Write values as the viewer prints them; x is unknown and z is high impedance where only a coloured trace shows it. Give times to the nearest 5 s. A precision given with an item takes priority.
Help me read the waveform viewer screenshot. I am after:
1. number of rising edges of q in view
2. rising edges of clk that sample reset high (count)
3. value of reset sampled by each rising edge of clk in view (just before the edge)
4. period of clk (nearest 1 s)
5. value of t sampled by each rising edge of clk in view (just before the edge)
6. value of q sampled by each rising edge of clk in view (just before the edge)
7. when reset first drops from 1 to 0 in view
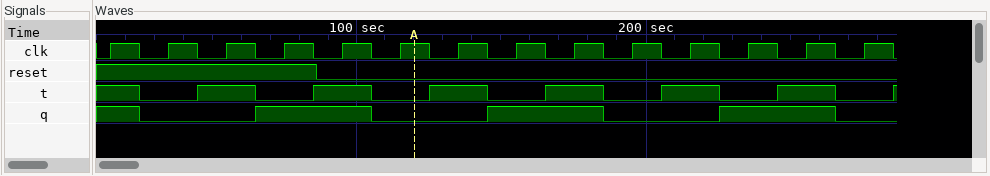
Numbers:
3
4
1 1 1 1 0 0 0 0 0 0 0 0 0 0
20 s
1 0 1 0 1 0 1 0 1 0 1 0 1 0
1 0 0 1 1 0 0 1 1 0 0 1 1 0
85 s
